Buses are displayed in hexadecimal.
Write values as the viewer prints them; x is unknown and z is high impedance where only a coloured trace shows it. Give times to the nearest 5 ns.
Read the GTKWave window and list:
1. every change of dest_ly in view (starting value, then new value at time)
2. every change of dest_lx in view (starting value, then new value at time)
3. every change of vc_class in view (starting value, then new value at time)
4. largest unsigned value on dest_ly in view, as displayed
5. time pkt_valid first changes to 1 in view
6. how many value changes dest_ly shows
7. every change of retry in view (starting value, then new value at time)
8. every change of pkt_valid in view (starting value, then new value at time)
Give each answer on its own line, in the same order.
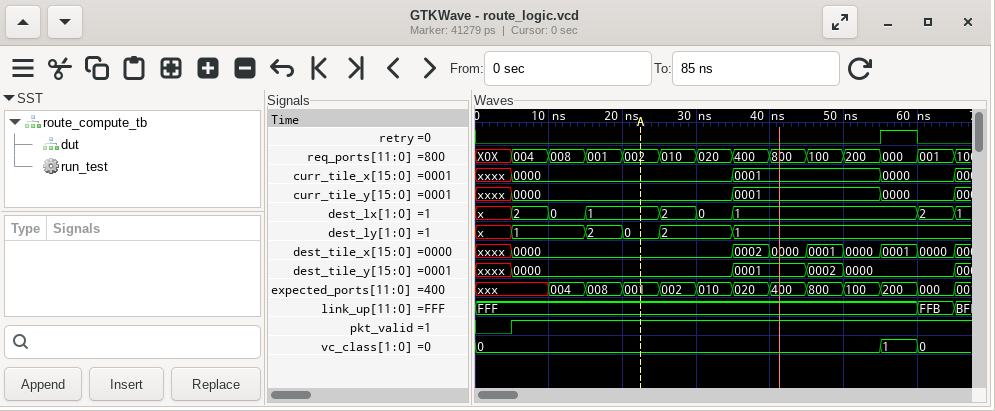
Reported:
x, 1 at 5 ns, 2 at 15 ns, 0 at 20 ns, 2 at 25 ns, 1 at 35 ns
x, 2 at 5 ns, 0 at 10 ns, 1 at 15 ns, 2 at 25 ns, 0 at 30 ns, 1 at 35 ns, 2 at 60 ns, 1 at 65 ns
0, 1 at 55 ns, 0 at 60 ns
2
5 ns
5
0, 1 at 55 ns, 0 at 60 ns
0, 1 at 5 ns
